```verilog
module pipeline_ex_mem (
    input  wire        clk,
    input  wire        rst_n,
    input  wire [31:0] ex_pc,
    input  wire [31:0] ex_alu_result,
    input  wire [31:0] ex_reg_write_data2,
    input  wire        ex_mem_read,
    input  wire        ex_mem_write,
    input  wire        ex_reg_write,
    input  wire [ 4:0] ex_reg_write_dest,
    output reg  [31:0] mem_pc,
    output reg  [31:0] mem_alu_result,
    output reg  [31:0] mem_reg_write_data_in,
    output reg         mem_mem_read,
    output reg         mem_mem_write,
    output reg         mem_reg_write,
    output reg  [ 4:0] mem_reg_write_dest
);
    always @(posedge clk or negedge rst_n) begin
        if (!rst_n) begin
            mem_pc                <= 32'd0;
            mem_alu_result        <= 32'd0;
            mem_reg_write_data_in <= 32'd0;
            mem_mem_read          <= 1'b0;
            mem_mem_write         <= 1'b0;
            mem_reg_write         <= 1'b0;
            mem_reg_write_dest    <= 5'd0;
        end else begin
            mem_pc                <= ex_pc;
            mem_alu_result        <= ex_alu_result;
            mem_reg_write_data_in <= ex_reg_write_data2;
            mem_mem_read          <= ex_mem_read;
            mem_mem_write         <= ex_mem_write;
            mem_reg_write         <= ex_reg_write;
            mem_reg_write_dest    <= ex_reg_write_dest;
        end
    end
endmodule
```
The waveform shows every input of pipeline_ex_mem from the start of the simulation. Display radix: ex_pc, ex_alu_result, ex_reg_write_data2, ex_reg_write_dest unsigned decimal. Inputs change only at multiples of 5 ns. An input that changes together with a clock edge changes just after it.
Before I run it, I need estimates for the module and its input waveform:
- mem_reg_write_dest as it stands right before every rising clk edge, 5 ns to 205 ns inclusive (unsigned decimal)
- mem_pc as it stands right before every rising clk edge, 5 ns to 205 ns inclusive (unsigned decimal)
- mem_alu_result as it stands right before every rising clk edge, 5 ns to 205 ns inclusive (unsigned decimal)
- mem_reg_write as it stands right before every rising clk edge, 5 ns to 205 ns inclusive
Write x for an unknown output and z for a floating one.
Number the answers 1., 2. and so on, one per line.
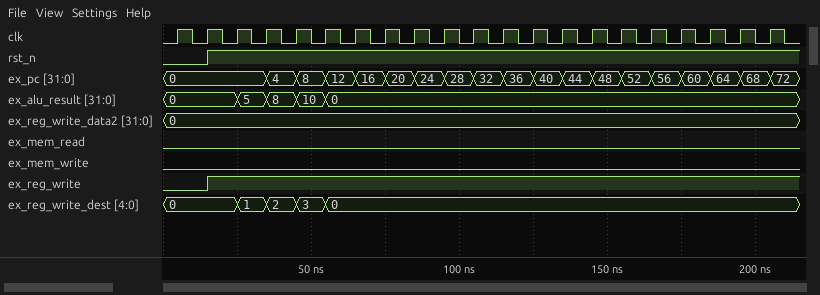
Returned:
1. 0, 0, 0, 0, 1, 2, 3, 0, 0, 0, 0, 0, 0, 0, 0, 0, 0, 0, 0, 0, 0
2. 0, 0, 0, 0, 0, 4, 8, 12, 16, 20, 24, 28, 32, 36, 40, 44, 48, 52, 56, 60, 64
3. 0, 0, 0, 0, 5, 8, 10, 0, 0, 0, 0, 0, 0, 0, 0, 0, 0, 0, 0, 0, 0
4. 0 0 0 1 1 1 1 1 1 1 1 1 1 1 1 1 1 1 1 1 1
